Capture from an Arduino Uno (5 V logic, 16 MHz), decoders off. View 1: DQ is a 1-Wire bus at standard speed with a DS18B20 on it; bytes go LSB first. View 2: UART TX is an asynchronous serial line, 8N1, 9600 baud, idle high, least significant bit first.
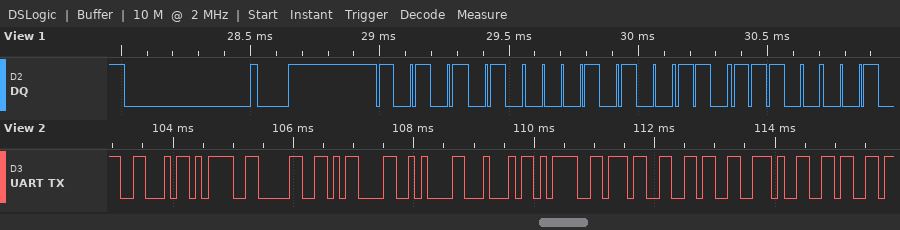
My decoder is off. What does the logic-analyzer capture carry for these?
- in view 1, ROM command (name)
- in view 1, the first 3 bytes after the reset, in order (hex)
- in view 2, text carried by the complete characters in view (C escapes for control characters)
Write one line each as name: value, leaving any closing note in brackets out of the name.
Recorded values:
in view 1, ROM command: Match ROM
in view 1, the first 3 bytes after the reset, in order: 55 28 3B
in view 2, text carried by the complete characters in view: "F=0\r\nD=76.6"
